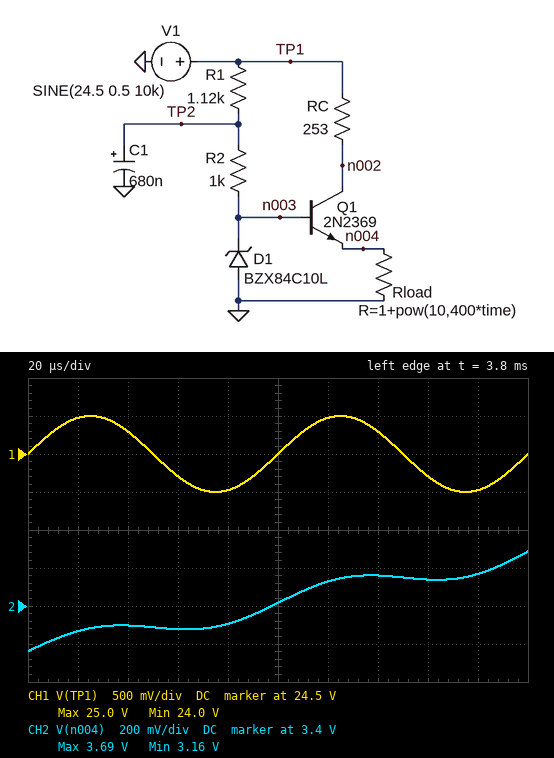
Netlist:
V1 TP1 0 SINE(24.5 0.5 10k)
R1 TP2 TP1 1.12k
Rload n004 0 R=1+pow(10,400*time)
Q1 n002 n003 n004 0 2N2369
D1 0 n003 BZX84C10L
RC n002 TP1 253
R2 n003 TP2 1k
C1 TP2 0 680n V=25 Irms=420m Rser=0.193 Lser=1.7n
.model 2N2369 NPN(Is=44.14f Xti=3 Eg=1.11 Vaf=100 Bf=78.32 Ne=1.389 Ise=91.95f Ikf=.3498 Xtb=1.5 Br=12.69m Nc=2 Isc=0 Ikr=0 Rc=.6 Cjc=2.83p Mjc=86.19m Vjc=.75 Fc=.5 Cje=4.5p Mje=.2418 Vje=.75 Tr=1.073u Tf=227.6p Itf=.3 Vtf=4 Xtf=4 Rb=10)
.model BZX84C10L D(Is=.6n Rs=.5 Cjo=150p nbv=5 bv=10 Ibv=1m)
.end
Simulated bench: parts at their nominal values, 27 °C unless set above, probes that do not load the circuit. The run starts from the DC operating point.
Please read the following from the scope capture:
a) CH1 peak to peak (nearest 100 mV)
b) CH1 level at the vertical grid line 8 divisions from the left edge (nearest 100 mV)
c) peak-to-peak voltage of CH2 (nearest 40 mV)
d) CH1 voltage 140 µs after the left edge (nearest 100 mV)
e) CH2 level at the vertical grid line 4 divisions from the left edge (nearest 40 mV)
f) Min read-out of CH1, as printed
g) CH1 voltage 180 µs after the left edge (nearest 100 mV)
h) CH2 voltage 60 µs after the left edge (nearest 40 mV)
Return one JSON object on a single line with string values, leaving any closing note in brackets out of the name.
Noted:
{"CH1 peak to peak": "1.0 V", "CH1 level at the vertical grid line 8 divisions from the left edge": "24.2 V", "peak-to-peak voltage of CH2": "520 mV", "CH1 voltage 140 µs after the left edge": "24.8 V", "CH2 level at the vertical grid line 4 divisions from the left edge": "3.32 V", "Min read-out of CH1, as printed": "24.0 V", "CH1 voltage 180 µs after the left edge": "24.0 V", "CH2 voltage 60 µs after the left edge": "3.28 V"}
